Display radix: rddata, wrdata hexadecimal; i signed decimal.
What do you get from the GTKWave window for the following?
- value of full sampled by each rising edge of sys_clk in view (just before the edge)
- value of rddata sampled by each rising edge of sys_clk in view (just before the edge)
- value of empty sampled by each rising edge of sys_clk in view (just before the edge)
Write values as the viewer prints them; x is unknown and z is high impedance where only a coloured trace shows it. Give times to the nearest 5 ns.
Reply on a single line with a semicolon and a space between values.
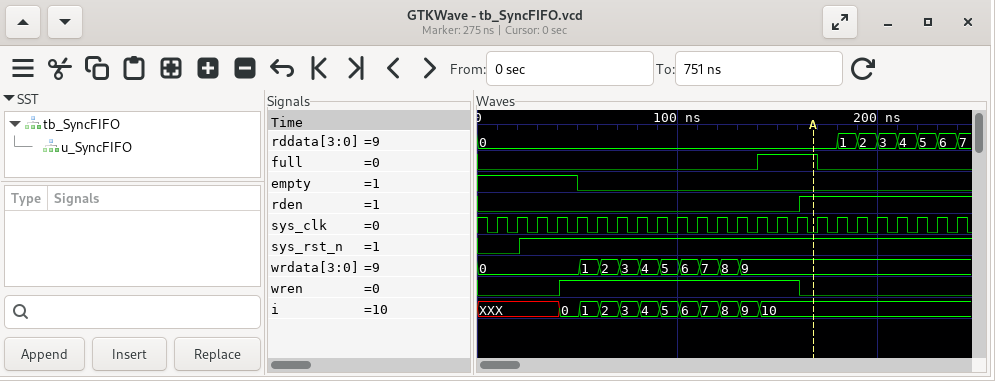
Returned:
0 0 0 0 0 0 0 0 0 0 0 0 0 0 1 1 1 0 0 0 0 0 0 0; 0, 0, 0, 0, 0, 0, 0, 0, 0, 0, 0, 0, 0, 0, 0, 0, 0, 0, 1, 2, 3, 4, 5, 6; 1 1 1 1 1 0 0 0 0 0 0 0 0 0 0 0 0 0 0 0 0 0 0 0
